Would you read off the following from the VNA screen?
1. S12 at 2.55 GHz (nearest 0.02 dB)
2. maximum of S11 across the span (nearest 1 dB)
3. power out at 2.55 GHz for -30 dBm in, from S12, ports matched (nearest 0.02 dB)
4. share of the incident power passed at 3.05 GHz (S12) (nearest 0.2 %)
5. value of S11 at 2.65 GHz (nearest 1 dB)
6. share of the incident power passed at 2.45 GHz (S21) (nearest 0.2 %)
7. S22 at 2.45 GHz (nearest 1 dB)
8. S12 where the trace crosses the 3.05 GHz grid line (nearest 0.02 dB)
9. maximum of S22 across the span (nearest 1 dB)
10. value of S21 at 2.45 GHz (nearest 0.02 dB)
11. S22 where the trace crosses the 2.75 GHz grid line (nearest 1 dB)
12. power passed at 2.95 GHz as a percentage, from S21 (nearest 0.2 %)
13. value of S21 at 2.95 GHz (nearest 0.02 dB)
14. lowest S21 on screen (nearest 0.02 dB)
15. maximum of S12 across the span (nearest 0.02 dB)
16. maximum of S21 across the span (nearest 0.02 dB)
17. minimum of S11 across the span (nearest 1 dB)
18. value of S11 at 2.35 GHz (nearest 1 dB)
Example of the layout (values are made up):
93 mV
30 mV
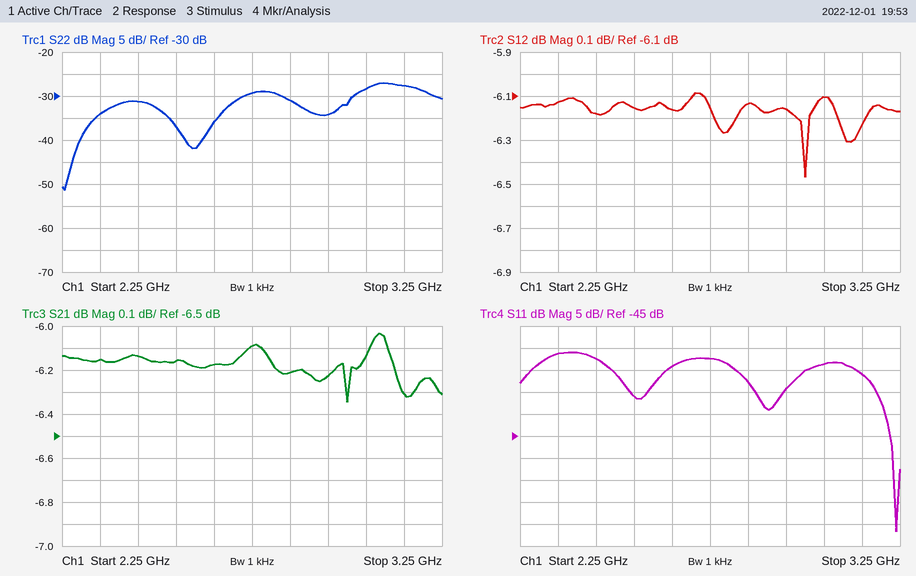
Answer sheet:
-6.16 dB
-26 dB
-36.16 dBm
24.6 %
-29 dB
24.4 %
-31 dB
-6.10 dB
-27 dB
-6.14 dB
-29 dB
23.8 %
-6.22 dB
-6.34 dB
-6.08 dB
-6.04 dB
-67 dB
-26 dB
